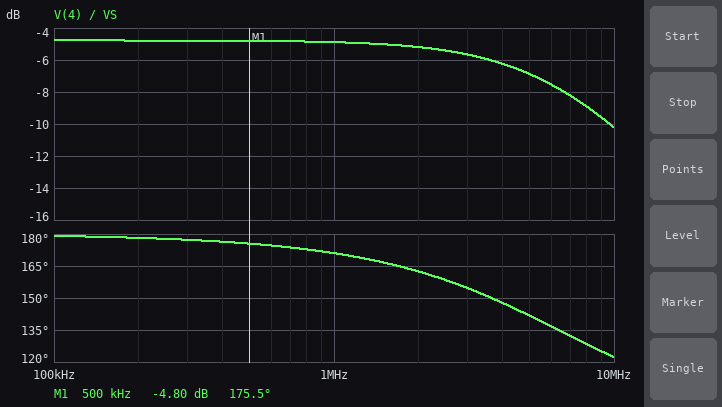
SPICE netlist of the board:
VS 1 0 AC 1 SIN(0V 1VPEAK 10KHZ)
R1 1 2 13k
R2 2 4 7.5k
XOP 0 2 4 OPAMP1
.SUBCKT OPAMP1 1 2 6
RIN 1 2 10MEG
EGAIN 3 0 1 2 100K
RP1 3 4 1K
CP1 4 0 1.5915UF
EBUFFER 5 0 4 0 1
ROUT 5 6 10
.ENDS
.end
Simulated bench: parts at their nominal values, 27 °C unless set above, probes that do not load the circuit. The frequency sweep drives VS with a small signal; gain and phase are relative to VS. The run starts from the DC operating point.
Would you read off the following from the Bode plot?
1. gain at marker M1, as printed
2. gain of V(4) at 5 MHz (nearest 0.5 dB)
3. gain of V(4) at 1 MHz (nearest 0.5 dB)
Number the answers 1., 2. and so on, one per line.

1. -4.80 dB
2. -7.0 dB
3. -5.0 dB
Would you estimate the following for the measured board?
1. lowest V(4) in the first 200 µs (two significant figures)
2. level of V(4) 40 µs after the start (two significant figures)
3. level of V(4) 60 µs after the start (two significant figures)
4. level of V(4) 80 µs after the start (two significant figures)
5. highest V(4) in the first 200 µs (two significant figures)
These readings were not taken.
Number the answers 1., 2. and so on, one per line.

1. -580 mV
2. -340 mV
3. 340 mV
4. 550 mV
5. 580 mV
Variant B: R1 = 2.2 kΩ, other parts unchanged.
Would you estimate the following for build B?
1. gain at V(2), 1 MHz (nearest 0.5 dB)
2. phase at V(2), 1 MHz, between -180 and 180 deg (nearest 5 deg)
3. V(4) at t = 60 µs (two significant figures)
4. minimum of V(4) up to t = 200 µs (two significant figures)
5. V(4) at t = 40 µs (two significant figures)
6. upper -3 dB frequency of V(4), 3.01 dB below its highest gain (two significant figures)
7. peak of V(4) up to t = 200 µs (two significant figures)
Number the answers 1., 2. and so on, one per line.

1. -10.0 dB
2. 65 deg
3. 2.0 V
4. -3.4 V
5. -2.0 V
6. 2.3 MHz
7. 3.4 V
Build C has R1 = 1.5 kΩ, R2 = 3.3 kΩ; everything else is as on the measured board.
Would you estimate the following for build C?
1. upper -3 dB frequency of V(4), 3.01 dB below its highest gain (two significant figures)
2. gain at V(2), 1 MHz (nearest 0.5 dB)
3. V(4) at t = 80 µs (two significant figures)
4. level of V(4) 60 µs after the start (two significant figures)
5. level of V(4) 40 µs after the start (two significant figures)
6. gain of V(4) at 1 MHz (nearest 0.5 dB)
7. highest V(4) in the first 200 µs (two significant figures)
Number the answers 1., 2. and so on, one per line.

1. 3.1 MHz
2. -13.5 dB
3. 2.1 V
4. 1.3 V
5. -1.3 V
6. 6.5 dB
7. 2.2 V
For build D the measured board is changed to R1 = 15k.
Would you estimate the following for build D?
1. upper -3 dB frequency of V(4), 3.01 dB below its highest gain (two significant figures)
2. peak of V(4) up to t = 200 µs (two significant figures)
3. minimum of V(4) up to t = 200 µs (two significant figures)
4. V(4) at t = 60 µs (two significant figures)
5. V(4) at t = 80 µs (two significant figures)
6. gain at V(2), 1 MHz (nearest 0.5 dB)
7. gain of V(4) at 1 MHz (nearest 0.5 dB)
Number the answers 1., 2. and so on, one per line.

1. 6.7 MHz
2. 500 mV
3. -500 mV
4. 290 mV
5. 480 mV
6. -26.0 dB
7. -6.0 dB
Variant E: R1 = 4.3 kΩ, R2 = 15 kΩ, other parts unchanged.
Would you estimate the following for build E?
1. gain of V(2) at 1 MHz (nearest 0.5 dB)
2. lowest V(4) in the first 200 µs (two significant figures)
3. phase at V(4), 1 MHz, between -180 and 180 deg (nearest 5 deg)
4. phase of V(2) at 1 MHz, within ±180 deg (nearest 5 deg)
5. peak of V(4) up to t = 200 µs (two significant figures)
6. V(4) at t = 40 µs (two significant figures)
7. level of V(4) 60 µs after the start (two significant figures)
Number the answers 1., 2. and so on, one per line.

1. -10.0 dB
2. -3.5 V
3. 155 deg
4. 65 deg
5. 3.5 V
6. -2.1 V
7. 2.0 V
